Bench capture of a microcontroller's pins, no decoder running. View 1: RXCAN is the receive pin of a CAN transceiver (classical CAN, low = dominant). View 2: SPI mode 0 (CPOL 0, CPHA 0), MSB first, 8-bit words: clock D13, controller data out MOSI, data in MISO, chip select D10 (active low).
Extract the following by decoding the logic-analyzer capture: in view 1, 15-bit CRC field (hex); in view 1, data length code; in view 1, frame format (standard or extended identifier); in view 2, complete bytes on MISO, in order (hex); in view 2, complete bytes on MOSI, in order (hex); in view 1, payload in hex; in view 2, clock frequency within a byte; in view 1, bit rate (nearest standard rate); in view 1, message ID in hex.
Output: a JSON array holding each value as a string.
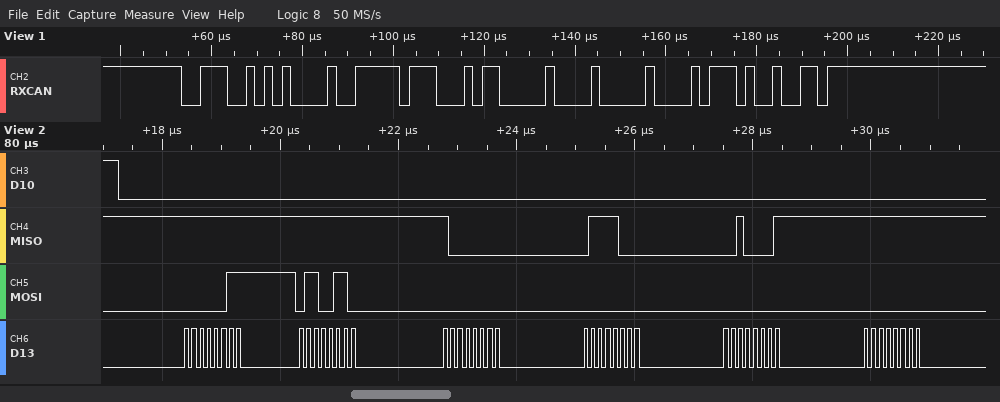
["0x1749", "4", "standard", "FF FF 80 78 21 FF", "03 66 00 00 00 00", "FF 16 00 80", "8 MHz", "500 kbit/s", "0x395"]
